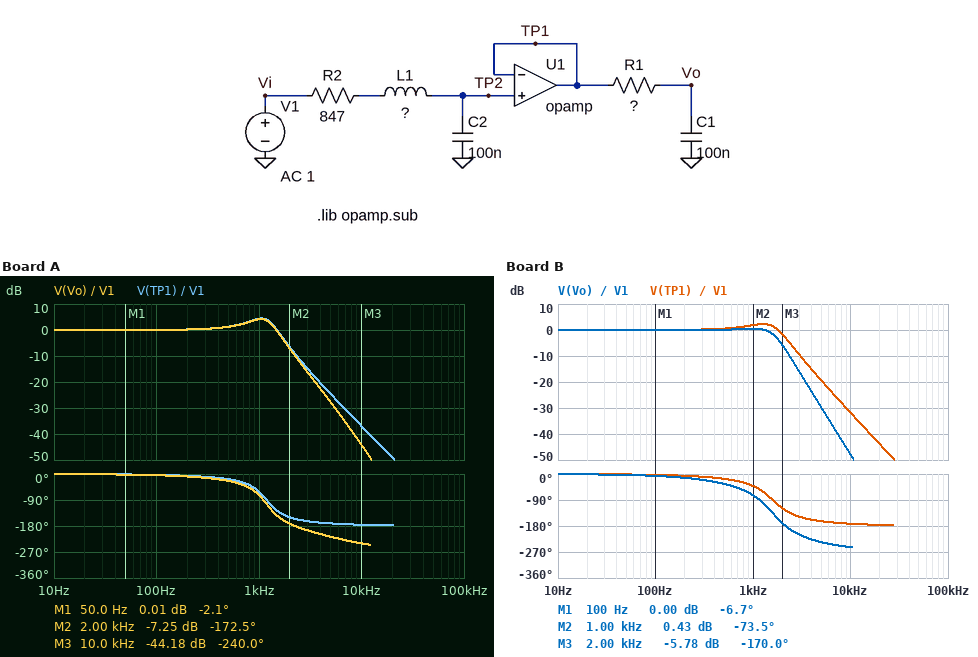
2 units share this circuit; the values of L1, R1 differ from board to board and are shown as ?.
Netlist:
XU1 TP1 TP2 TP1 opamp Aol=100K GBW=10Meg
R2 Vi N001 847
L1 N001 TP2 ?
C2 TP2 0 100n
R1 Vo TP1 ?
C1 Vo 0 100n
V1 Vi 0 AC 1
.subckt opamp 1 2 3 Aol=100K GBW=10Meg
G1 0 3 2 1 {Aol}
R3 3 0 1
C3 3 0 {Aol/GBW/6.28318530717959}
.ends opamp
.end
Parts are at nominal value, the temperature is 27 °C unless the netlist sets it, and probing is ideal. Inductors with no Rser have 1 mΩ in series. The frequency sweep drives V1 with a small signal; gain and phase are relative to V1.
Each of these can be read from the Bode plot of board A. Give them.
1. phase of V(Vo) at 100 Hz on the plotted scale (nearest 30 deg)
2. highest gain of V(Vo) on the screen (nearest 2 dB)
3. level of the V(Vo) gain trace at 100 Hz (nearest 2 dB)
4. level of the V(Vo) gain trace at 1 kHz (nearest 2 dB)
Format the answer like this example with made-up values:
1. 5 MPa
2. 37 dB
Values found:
1. 0 deg
2. 4 dB
3. 0 dB
4. 4 dB
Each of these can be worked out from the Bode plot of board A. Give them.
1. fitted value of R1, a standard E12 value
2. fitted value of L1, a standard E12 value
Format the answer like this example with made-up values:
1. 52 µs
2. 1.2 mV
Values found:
1. 330 Ω
2. 180 mH
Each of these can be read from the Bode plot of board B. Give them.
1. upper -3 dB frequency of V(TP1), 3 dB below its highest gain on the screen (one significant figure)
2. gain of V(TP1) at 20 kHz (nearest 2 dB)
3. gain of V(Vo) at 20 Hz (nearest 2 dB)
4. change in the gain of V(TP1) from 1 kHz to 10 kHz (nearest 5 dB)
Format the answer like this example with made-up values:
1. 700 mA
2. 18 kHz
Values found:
1. 2 kHz
2. -44 dB
3. 0 dB
4. -35 dB
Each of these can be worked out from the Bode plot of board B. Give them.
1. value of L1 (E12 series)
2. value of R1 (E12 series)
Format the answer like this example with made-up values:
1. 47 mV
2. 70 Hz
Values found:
1. 100 mH
2. 1 kΩ
